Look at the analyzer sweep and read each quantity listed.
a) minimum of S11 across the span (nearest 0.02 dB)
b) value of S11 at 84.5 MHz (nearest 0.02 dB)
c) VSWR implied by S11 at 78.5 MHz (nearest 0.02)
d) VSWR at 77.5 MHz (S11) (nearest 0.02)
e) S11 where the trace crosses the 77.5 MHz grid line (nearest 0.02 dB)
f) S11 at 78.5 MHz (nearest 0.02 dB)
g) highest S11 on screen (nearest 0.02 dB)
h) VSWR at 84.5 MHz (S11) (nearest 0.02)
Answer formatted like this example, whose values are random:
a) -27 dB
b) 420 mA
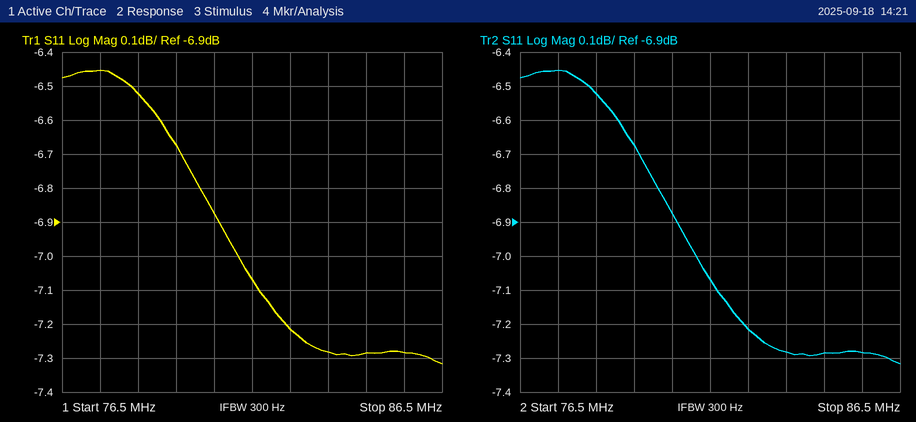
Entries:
a) -7.32 dB
b) -7.28 dB
c) 2.78
d) 2.82
e) -6.46 dB
f) -6.52 dB
g) -6.46 dB
h) 2.52
